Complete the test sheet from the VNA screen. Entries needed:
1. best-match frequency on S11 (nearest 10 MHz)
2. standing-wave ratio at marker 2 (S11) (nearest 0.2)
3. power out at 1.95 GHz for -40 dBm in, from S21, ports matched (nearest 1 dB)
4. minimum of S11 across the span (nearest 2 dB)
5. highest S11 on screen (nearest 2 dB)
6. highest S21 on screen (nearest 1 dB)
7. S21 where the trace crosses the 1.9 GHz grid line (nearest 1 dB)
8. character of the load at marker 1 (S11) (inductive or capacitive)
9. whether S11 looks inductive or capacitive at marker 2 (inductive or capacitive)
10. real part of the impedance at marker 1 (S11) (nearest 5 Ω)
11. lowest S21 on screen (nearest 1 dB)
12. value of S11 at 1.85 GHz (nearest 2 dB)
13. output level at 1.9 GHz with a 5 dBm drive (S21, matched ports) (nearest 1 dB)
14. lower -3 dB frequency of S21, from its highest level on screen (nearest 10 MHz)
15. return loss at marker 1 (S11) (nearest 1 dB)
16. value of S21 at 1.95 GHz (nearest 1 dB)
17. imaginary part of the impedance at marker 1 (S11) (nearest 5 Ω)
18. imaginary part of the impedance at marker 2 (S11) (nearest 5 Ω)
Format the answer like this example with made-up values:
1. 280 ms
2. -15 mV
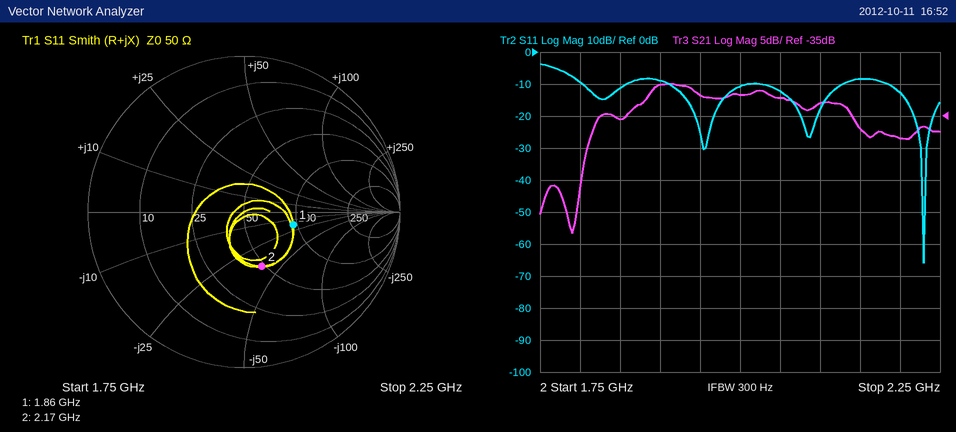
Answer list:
1. 2.23 GHz
2. 2.2
3. -72 dBm
4. -66 dB
5. -4 dB
6. -30 dB
7. -30 dB
8. capacitive
9. capacitive
10. 95 Ω
11. -53 dB
12. -12 dB
13. -25 dBm
14. 1.88 GHz
15. 10 dB
16. -32 dB
17. -15 Ω
18. -40 Ω
